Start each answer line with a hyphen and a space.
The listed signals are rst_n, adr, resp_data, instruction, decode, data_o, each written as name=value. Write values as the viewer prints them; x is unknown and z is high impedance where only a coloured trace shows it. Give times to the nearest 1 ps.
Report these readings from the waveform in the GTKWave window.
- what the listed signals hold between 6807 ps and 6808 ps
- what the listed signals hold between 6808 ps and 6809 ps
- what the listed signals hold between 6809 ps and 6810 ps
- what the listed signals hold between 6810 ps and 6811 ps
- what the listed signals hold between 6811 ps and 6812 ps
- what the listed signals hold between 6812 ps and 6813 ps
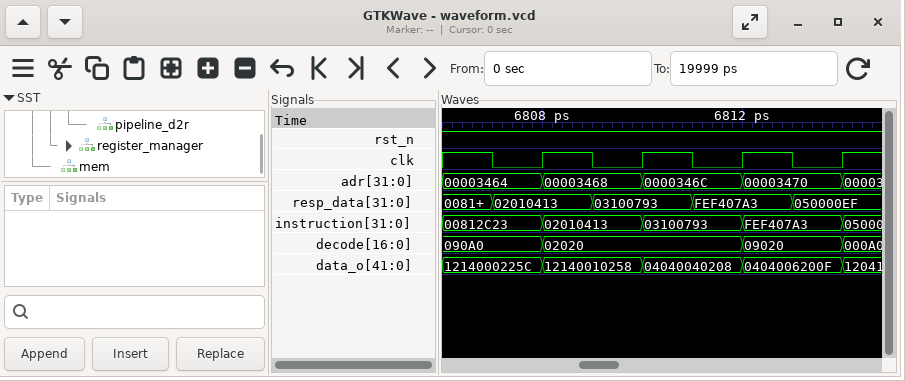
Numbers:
- rst_n=1, adr=00003464, resp_data=02010413, instruction=00812C23, decode=090A0, data_o=1214000225C
- rst_n=1, adr=00003468, resp_data=02010413, instruction=02010413, decode=02020, data_o=12140010258
- rst_n=1, adr=00003468, resp_data=03100793, instruction=02010413, decode=02020, data_o=12140010258
- rst_n=1, adr=0000346C, resp_data=03100793, instruction=03100793, decode=02020, data_o=04040040208
- rst_n=1, adr=0000346C, resp_data=FEF407A3, instruction=03100793, decode=02020, data_o=04040040208
- rst_n=1, adr=00003470, resp_data=FEF407A3, instruction=FEF407A3, decode=09020, data_o=0404006200F
